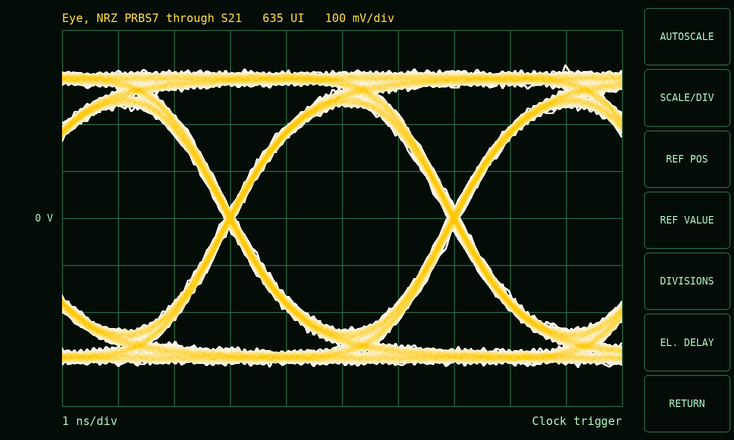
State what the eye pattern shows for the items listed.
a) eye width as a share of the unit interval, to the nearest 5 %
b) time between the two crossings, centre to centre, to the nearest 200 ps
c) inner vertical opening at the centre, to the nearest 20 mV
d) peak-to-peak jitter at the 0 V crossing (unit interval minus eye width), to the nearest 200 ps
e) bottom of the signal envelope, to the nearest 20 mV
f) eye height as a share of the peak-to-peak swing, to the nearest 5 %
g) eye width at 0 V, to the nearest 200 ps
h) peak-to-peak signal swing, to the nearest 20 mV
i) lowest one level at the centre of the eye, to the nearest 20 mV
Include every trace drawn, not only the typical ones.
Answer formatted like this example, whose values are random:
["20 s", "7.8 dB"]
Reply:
["95 %", "4.0 ns", "480 mV", "200 ps", "-320 mV", "75 %", "3.8 ns", "640 mV", "240 mV"]
